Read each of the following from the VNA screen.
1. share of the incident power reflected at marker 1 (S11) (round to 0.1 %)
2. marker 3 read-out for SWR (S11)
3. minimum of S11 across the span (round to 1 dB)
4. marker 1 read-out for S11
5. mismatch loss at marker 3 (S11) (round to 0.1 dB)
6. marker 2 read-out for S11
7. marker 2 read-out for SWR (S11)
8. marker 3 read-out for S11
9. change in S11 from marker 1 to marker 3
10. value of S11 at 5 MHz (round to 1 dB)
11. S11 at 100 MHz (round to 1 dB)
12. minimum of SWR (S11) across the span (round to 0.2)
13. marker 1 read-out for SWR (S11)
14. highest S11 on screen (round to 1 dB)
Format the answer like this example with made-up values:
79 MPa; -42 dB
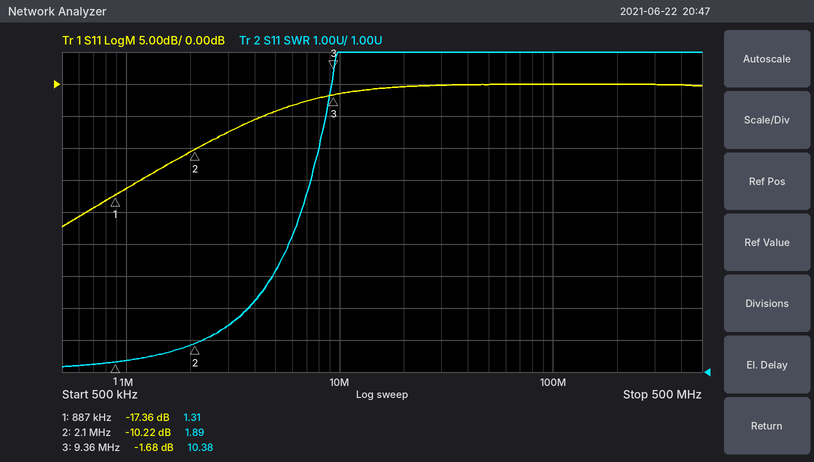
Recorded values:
1.8 %; 10.38; -22 dB; -17.36 dB; 4.9 dB; -10.22 dB; 1.89; -1.68 dB; 15.68 dB; -4 dB; 0 dB; 1.2; 1.31; 0 dB
